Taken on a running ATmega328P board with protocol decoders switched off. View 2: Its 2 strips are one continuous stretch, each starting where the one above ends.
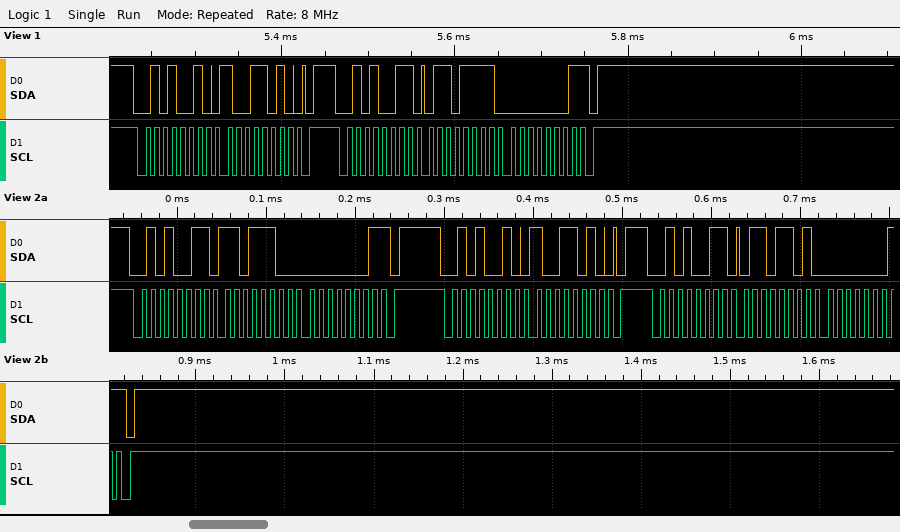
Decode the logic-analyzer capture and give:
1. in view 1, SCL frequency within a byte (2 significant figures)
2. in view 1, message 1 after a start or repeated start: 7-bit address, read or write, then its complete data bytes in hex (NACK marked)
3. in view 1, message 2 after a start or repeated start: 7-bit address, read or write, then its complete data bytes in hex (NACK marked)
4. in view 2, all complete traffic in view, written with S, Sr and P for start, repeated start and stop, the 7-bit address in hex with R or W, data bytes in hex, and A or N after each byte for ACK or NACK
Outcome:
100 kHz
0x29 write: 9A
0x29 read: 6F 01 NACK
S 29R A DC A 01 N P S 29W A 9A A P S 29R A 6D A 01 N P
